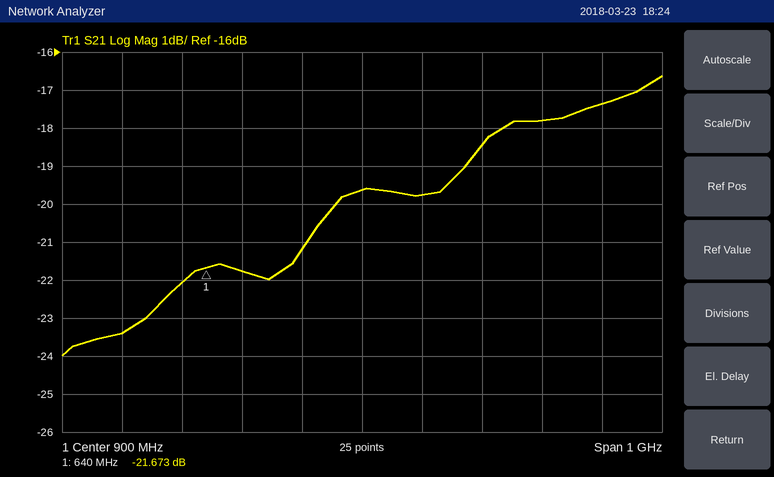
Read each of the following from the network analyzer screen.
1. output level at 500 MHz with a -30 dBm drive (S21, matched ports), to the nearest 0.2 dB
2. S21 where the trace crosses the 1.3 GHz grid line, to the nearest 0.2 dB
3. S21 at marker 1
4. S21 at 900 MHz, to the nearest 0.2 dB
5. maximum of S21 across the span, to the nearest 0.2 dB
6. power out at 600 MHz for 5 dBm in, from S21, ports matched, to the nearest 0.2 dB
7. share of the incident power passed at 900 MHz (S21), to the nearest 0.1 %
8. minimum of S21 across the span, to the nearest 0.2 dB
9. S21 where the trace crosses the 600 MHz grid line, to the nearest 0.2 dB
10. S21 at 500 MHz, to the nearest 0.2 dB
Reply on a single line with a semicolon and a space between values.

-53.4 dBm; -17.4 dB; -21.673 dB; -19.6 dB; -16.6 dB; -17.0 dBm; 1.1 %; -24.0 dB; -22.0 dB; -23.4 dB
